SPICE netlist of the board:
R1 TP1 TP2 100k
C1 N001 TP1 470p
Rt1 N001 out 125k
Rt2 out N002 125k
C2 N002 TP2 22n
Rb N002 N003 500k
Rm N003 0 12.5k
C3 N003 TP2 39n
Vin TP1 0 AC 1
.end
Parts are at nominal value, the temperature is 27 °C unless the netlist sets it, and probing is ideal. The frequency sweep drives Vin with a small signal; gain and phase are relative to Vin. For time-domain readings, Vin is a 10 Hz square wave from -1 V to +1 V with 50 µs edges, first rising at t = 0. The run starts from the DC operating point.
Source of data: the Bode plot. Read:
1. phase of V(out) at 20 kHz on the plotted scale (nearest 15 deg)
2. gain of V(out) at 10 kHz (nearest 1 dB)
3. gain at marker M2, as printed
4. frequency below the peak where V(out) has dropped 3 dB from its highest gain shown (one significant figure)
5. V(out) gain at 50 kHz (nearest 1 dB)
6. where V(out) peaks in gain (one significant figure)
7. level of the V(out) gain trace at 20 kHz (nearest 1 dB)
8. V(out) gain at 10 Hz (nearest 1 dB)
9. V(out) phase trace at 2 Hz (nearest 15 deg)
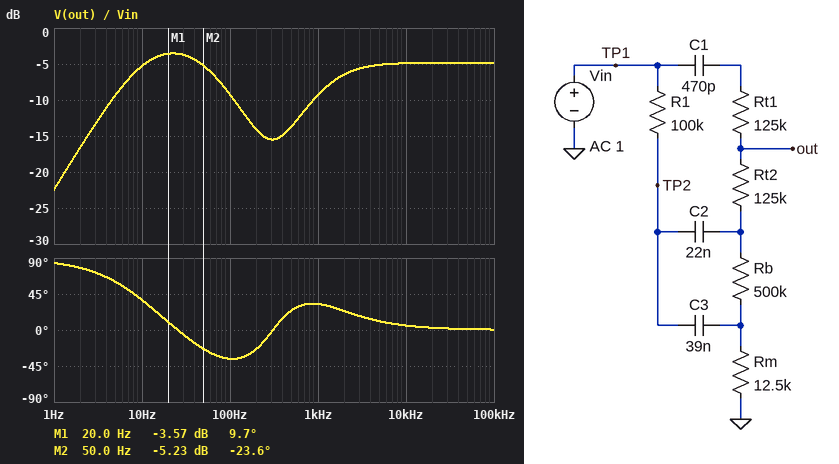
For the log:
0 deg
-5 dB
-5.23 dB
8 Hz
-5 dB
20 Hz
-5 dB
-5 dB
75 deg
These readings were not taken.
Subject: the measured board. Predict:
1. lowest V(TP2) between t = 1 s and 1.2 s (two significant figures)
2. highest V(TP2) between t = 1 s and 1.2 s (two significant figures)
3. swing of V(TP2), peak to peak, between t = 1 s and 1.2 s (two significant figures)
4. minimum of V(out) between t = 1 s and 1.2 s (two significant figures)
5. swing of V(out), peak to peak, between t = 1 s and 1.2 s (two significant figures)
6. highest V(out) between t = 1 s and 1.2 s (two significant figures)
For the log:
-980 mV
980 mV
2.0 V
-1.0 V
2.0 V
1.0 V
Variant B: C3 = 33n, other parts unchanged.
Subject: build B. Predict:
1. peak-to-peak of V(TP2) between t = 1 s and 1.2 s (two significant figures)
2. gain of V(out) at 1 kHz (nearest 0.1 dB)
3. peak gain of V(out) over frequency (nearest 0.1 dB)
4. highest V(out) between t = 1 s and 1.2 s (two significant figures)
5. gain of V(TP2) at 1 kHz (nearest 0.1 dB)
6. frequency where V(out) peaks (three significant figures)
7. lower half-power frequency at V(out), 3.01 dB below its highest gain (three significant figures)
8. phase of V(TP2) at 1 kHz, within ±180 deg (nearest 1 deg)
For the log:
2.0 V
-9.4 dB
-3.3 dB
1.1 V
-17.4 dB
24.4 Hz
8.12 Hz
-10 deg
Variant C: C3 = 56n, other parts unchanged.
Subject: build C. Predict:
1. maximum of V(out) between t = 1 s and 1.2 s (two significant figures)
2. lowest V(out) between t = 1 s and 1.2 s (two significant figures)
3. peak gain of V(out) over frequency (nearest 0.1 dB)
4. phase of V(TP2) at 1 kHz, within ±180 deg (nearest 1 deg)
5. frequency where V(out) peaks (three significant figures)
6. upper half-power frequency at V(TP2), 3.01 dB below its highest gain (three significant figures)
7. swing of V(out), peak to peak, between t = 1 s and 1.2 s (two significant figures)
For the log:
910 mV
-910 mV
-4.2 dB
-3 deg
18.9 Hz
19.4 Hz
1.8 V
